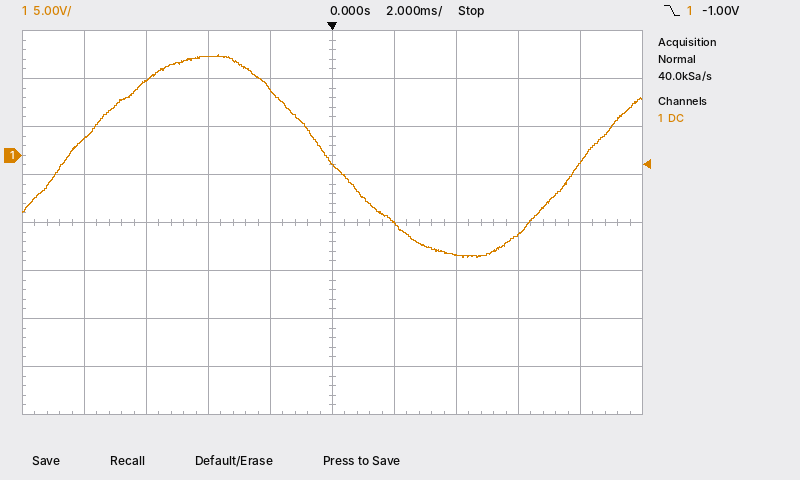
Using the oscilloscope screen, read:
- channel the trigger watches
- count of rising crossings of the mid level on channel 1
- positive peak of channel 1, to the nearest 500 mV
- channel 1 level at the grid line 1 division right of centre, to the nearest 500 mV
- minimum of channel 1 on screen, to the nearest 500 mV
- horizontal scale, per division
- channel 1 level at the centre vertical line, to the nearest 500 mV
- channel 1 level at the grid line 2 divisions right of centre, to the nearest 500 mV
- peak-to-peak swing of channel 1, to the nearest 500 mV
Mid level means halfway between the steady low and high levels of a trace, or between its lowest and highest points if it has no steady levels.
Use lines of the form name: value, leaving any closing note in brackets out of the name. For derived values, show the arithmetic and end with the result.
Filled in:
channel the trigger watches: channel 1
count of rising crossings of the mid level on channel 1: 2
positive peak of channel 1, to the nearest 500 mV: 10.5 V
channel 1 level at the grid line 1 division right of centre, to the nearest 500 mV: -7.0 V
minimum of channel 1 on screen, to the nearest 500 mV: -10.5 V
horizontal scale, per division: 2 ms
channel 1 level at the centre vertical line, to the nearest 500 mV: -1.0 V
channel 1 level at the grid line 2 divisions right of centre, to the nearest 500 mV: -10.5 V
peak-to-peak swing of channel 1, to the nearest 500 mV: 10.5 V − (-10.5 V) = 21.0 V
